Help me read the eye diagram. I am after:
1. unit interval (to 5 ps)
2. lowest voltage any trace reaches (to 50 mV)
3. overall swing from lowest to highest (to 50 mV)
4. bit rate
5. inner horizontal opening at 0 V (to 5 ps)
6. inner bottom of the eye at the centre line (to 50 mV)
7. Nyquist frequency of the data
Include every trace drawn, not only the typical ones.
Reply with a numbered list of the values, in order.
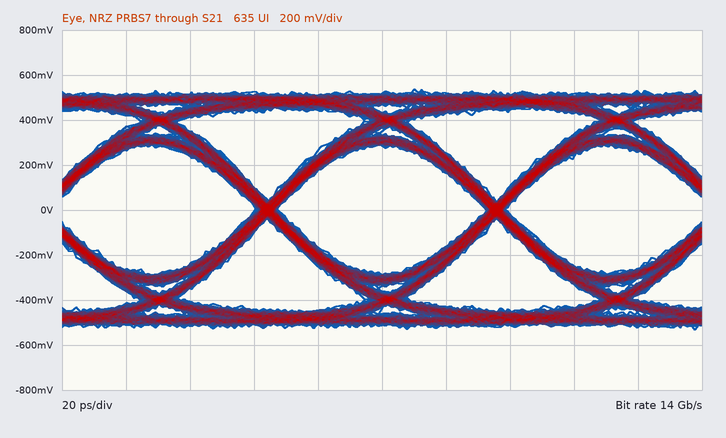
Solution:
1. 70 ps
2. -550 mV
3. 1.05 V
4. 14 Gb/s
5. 65 ps
6. -300 mV
7. 7 GHz
